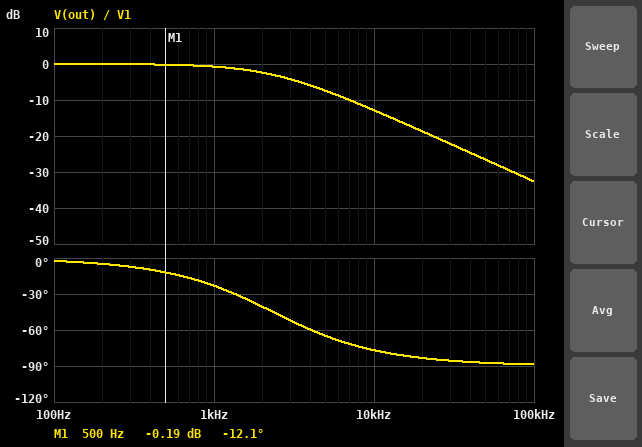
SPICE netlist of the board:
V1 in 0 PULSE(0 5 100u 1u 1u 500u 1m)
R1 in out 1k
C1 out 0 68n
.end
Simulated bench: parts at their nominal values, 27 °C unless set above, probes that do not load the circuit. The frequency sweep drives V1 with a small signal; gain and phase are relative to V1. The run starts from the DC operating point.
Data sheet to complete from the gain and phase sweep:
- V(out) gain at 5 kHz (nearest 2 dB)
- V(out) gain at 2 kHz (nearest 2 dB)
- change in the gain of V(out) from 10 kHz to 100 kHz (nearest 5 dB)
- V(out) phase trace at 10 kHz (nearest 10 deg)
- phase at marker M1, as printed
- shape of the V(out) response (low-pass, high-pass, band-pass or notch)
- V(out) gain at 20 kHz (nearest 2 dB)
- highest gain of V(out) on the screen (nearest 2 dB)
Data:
-8 dB
-2 dB
-20 dB
-80 deg
-12.1 deg
low-pass
-18 dB
0 dB
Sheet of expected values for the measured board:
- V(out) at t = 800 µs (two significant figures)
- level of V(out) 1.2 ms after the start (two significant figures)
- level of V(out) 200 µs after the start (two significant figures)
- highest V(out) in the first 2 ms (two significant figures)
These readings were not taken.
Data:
270 mV
3.8 V
3.8 V
5.0 V
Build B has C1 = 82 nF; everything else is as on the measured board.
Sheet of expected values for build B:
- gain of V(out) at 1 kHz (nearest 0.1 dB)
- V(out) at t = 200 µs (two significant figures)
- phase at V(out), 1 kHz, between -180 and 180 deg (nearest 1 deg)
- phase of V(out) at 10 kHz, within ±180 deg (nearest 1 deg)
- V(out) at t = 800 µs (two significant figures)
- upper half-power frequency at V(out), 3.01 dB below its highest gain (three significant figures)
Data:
-1.0 dB
3.5 V
-27 deg
-79 deg
440 mV
1.94 kHz
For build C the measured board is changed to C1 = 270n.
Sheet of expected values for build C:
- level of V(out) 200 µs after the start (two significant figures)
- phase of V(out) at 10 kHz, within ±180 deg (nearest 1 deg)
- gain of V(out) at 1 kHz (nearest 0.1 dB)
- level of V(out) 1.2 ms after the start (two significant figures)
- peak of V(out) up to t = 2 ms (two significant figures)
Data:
1.5 V
-87 deg
-5.9 dB
2.0 V
4.3 V
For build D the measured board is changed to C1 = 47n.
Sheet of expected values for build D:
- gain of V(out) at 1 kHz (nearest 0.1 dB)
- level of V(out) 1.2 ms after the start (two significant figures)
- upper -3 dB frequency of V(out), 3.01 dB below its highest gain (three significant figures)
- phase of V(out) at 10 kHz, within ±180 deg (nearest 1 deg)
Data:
-0.4 dB
4.4 V
3.39 kHz
-71 deg
